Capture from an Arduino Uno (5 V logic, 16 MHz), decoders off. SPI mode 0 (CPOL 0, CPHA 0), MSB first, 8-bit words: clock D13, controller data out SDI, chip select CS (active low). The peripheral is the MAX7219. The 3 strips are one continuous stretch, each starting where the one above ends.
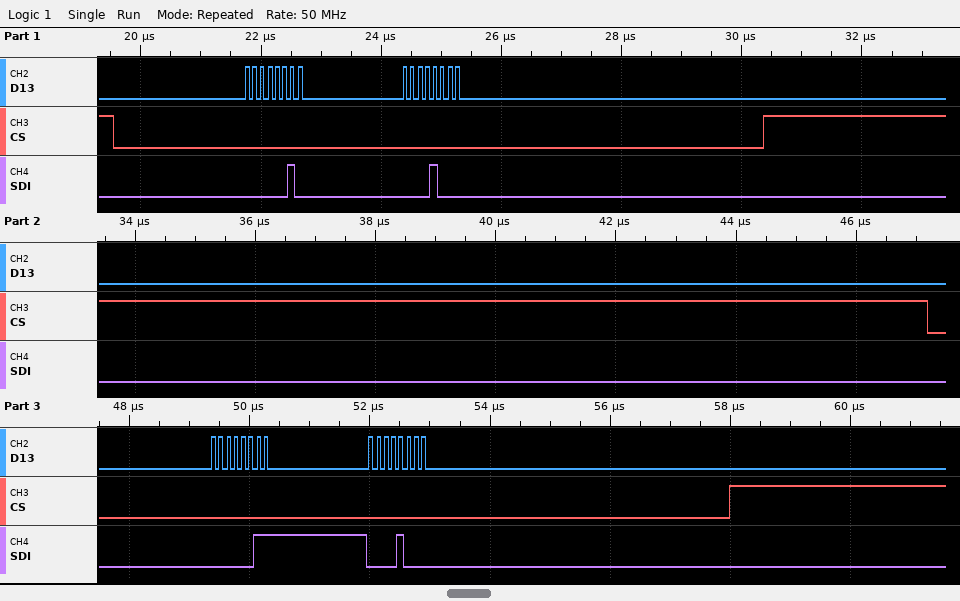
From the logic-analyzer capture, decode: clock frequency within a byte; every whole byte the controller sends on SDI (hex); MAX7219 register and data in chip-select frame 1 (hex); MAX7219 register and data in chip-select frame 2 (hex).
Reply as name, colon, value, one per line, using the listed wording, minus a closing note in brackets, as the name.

clock frequency within a byte: 8 MHz
every whole byte the controller sends on SDI: 02 08 03 08
MAX7219 register and data in chip-select frame 1: register 0x2, data 0x08
MAX7219 register and data in chip-select frame 2: register 0x3, data 0x08
